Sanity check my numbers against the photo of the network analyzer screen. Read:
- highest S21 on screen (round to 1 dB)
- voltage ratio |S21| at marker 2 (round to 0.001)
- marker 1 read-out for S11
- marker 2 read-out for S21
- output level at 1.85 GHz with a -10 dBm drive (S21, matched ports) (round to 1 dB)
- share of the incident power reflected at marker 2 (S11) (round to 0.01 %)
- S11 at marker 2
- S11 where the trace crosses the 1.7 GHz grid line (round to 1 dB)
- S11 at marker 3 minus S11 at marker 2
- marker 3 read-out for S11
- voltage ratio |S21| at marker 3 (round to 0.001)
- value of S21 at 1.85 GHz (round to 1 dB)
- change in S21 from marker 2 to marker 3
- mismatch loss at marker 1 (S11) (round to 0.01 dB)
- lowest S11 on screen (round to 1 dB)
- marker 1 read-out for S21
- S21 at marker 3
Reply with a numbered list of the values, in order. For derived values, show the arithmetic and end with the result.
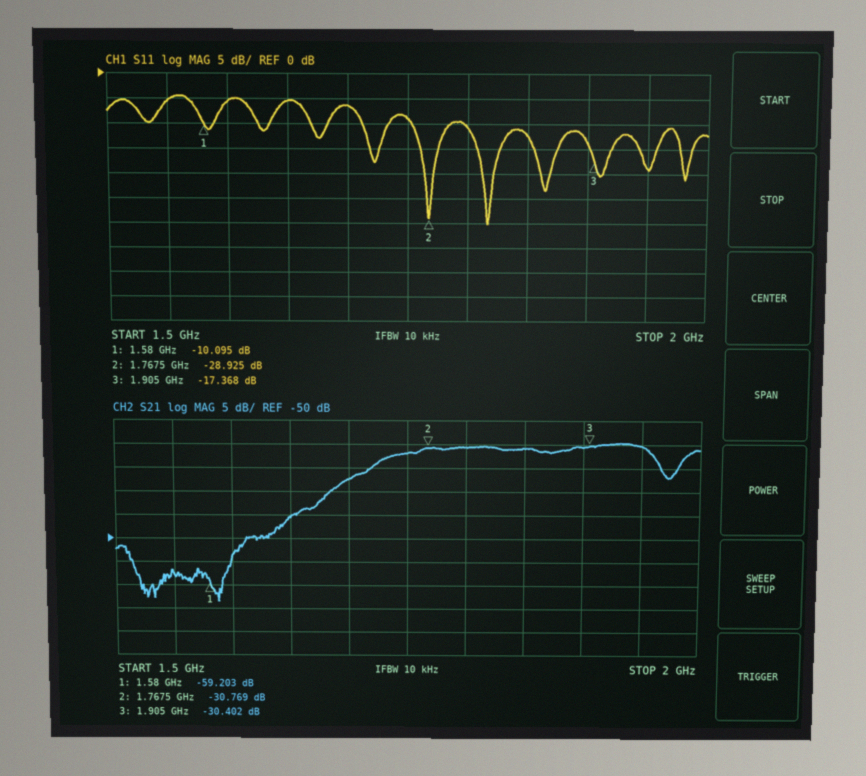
1. -30 dB
2. 10^(-30.769/20) ≈ 0.029
3. -10.095 dB
4. -30.769 dB
5. -10 dBm + (-31 dB) = -41 dBm
6. 10^(-28.925/10) ≈ 0.13 %
7. -28.925 dB
8. -6 dB
9. -17.368 − (-28.925) = 11.557 dB
10. -17.368 dB
11. 10^(-30.402/20) ≈ 0.030
12. -31 dB
13. -30.402 − (-30.769) = 0.367 dB
14. −10 log10(1 − 10^(-10.095/10)) ≈ 0.45 dB
15. -30 dB
16. -59.203 dB
17. -30.402 dB
